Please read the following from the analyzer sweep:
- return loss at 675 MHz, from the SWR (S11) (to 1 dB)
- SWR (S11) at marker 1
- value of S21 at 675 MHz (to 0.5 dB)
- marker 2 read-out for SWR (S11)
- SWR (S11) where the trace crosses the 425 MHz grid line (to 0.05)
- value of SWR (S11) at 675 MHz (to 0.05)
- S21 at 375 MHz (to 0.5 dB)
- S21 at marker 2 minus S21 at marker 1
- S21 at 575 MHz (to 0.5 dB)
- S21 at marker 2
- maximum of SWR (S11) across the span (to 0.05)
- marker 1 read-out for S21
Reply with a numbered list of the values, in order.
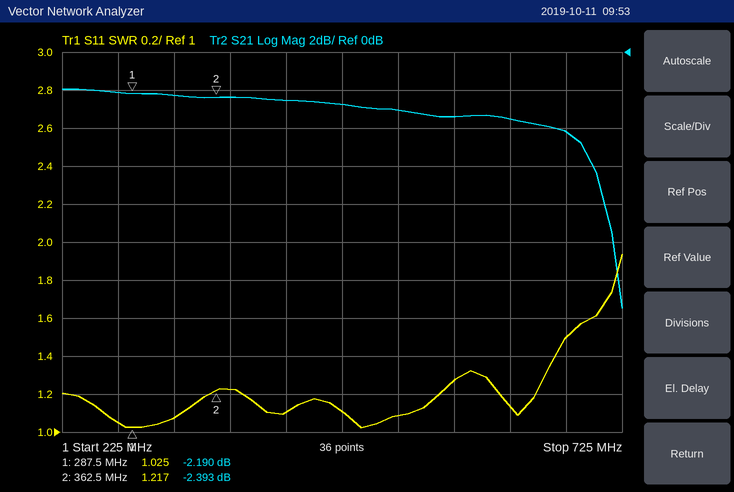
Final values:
1. 14 dB
2. 1.025
3. -4.0 dB
4. 1.217
5. 1.10
6. 1.50
7. -2.5 dB
8. -0.203 dB
9. -3.5 dB
10. -2.393 dB
11. 1.95
12. -2.190 dB
